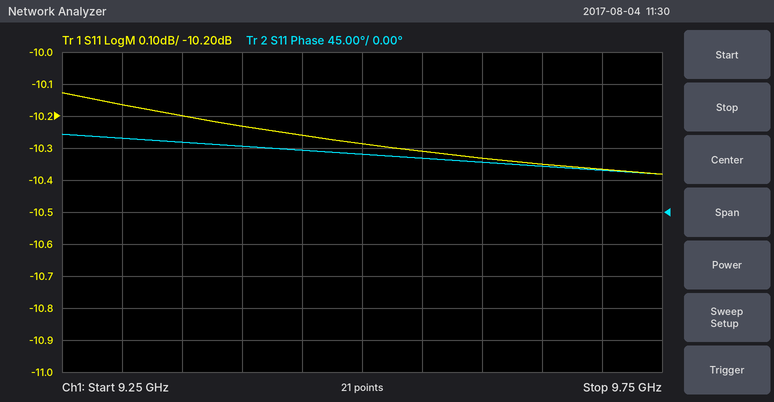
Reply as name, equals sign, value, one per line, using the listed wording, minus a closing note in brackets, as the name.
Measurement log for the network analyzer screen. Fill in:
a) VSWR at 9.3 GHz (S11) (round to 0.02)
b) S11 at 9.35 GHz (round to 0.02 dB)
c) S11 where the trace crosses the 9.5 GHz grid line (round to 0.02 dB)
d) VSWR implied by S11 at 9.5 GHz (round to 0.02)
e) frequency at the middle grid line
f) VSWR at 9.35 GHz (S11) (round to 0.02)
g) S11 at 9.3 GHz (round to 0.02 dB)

VSWR at 9.3 GHz (S11) = 1.90
S11 at 9.35 GHz = -10.20 dB
S11 where the trace crosses the 9.5 GHz grid line = -10.28 dB
VSWR implied by S11 at 9.5 GHz = 1.88
frequency at the middle grid line = 9.5 GHz
VSWR at 9.35 GHz (S11) = 1.90
S11 at 9.3 GHz = -10.16 dB
